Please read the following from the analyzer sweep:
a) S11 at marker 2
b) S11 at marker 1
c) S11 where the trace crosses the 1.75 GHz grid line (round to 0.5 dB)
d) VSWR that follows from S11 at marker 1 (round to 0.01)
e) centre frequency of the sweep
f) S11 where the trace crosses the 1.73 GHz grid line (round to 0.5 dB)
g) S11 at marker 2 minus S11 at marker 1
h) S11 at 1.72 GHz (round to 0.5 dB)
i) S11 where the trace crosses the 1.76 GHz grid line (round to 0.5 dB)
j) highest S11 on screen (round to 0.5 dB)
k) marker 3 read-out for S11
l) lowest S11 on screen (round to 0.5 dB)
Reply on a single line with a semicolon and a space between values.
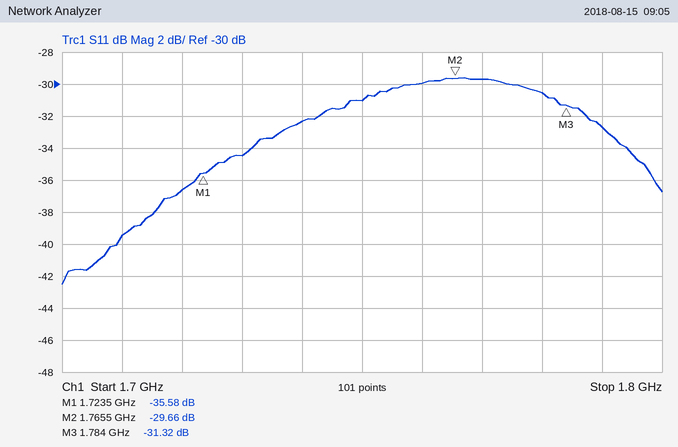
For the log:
-29.66 dB; -35.58 dB; -31.0 dB; 1.03; 1.75 GHz; -34.5 dB; 5.92 dB; -36.5 dB; -30.0 dB; -29.5 dB; -31.32 dB; -42.5 dB
